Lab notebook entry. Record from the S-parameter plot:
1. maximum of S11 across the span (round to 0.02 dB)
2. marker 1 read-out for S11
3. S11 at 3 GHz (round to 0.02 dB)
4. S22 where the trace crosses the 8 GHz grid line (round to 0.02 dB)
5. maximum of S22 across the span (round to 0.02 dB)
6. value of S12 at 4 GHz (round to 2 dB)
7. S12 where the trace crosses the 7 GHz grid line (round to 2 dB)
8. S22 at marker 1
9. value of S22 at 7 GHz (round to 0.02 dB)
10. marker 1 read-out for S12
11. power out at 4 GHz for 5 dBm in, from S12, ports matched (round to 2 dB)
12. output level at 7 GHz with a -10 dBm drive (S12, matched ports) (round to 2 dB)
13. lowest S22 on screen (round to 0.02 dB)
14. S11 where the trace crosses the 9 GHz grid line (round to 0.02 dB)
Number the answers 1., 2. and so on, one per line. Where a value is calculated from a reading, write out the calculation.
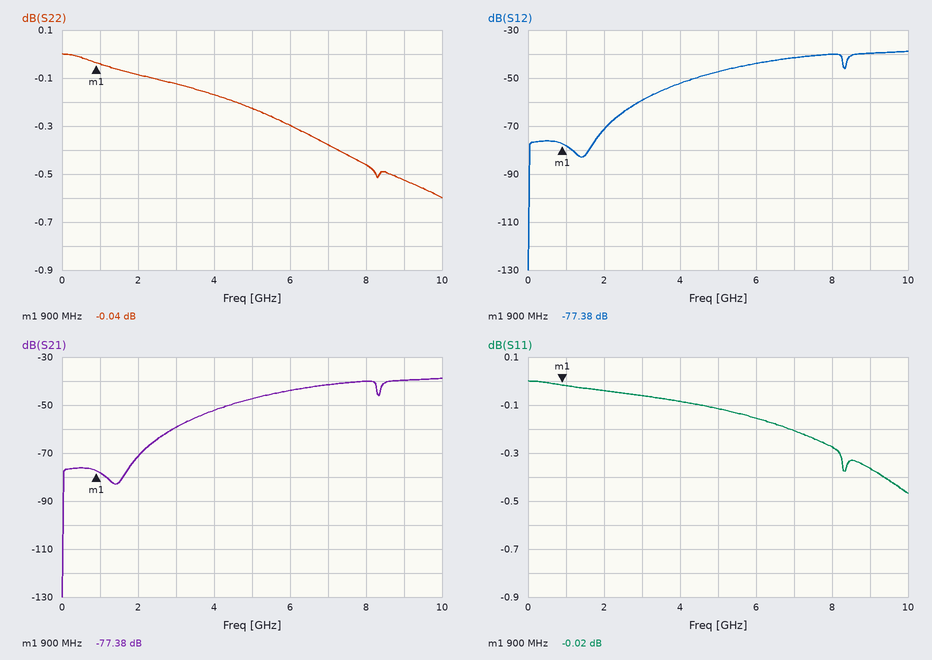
1. 0.00 dB
2. -0.02 dB
3. -0.06 dB
4. -0.46 dB
5. 0.00 dB
6. -52 dB
7. -42 dB
8. -0.04 dB
9. -0.38 dB
10. -77.38 dB
11. 5 dBm + (-52 dB) = -48 dBm
12. -10 dBm + (-42 dB) = -52 dBm
13. -0.60 dB
14. -0.36 dB
